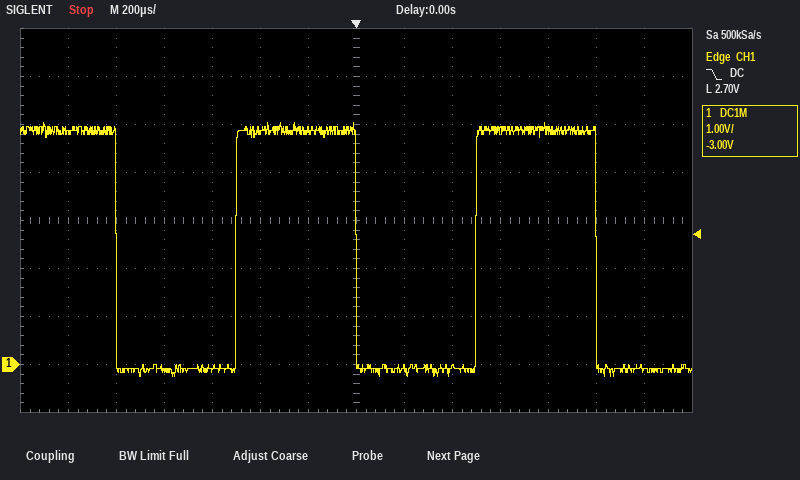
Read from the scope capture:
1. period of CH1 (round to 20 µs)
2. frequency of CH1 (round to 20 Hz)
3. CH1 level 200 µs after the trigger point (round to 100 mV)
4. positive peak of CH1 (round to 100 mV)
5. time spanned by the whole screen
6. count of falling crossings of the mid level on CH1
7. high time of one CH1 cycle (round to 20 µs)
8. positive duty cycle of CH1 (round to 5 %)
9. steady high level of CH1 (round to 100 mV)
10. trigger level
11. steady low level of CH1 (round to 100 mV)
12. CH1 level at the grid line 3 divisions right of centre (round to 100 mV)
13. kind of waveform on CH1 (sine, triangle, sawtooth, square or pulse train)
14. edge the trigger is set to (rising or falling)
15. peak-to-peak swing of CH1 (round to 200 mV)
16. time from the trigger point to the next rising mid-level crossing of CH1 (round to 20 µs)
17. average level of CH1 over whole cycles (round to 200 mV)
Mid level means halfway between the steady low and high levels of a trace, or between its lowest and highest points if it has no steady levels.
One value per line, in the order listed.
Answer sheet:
1.00 ms
1.00 kHz
-100 mV
5.0 V
2.8 ms
3
500 µs
50 %
4.9 V
2.70 V
-100 mV
4.9 V
square
falling
5.2 V
500 µs
2.4 V
